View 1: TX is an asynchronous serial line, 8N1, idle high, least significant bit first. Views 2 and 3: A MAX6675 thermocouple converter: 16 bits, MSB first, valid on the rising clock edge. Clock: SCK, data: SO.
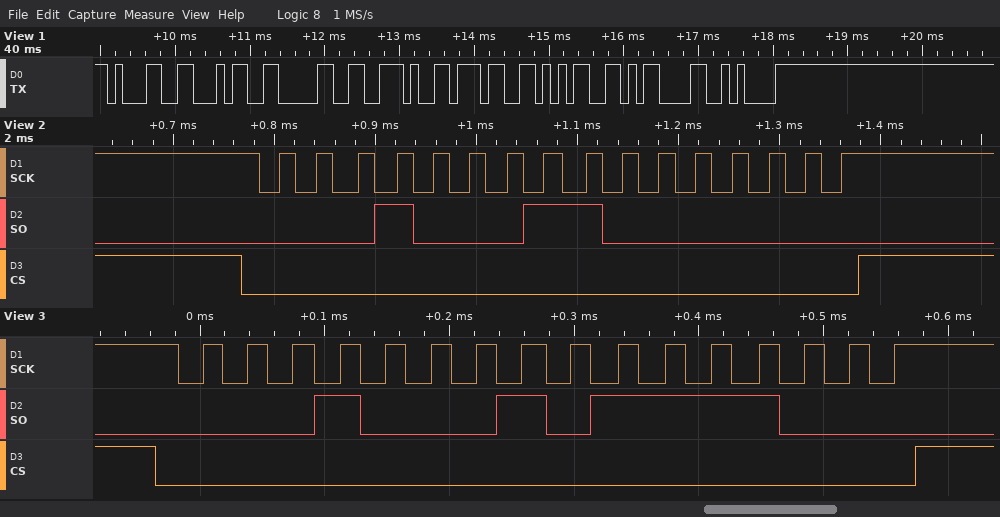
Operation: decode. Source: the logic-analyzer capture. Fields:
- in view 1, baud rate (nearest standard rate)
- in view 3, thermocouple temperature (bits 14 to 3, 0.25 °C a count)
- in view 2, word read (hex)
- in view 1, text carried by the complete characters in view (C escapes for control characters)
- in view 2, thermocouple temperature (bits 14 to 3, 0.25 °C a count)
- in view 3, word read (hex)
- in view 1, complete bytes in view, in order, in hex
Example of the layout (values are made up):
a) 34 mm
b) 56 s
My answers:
a) 9600 baud
b) 139.75 °C
c) 0x1180
d) "140.75\r\n"
e) 140.00 °C
f) 0x1178
g) 31 34 30 2E 37 35 0D 0A
